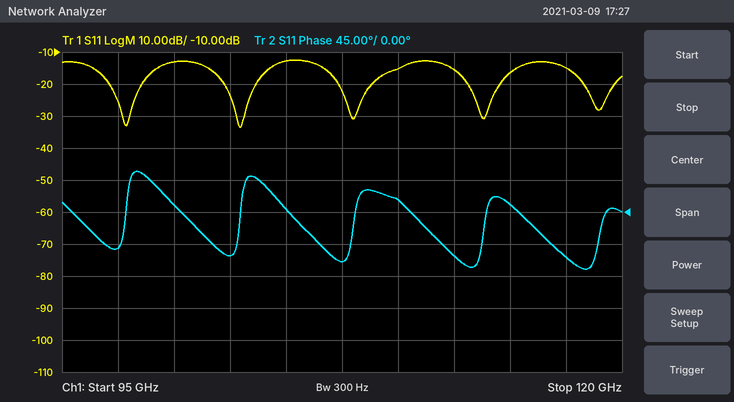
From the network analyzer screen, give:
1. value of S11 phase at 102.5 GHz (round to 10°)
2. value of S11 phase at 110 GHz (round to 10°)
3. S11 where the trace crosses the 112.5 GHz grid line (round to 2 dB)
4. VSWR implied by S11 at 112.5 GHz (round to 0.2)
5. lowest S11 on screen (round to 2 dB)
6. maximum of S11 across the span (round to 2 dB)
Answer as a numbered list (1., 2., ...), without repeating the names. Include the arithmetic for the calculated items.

1. -60°
2. 20°
3. -16 dB
4. |Γ| = 10^(-16/20) = 0.1585; VSWR = (1 + 0.1585)/(1 − 0.1585) ≈ 1.4
5. -34 dB
6. -12 dB
